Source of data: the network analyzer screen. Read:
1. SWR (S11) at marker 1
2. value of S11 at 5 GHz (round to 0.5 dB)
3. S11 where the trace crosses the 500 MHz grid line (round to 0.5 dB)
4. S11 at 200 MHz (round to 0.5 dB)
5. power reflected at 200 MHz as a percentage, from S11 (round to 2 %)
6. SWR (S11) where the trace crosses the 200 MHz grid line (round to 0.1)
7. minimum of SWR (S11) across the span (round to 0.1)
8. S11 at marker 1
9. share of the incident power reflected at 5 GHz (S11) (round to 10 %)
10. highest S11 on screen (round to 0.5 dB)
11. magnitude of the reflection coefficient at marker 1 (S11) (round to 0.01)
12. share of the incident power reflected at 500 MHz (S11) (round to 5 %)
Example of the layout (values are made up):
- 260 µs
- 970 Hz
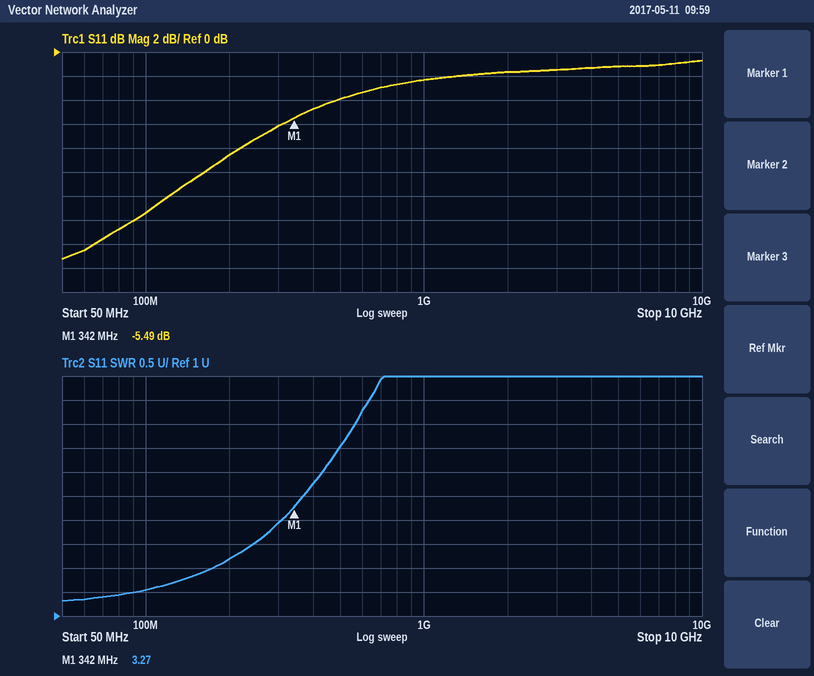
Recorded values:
- 3.27
- -1.0 dB
- -4.0 dB
- -8.5 dB
- 14 %
- 2.2
- 1.3
- -5.49 dB
- 80 %
- -0.5 dB
- 0.53
- 40 %
